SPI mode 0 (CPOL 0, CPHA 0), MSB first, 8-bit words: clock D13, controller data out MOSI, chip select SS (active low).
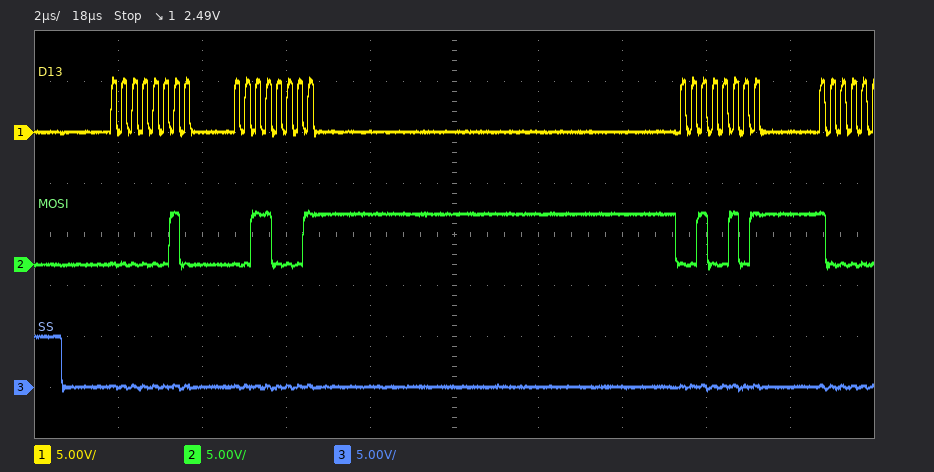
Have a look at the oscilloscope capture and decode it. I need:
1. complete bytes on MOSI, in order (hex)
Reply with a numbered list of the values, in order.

1. 02 31 25
